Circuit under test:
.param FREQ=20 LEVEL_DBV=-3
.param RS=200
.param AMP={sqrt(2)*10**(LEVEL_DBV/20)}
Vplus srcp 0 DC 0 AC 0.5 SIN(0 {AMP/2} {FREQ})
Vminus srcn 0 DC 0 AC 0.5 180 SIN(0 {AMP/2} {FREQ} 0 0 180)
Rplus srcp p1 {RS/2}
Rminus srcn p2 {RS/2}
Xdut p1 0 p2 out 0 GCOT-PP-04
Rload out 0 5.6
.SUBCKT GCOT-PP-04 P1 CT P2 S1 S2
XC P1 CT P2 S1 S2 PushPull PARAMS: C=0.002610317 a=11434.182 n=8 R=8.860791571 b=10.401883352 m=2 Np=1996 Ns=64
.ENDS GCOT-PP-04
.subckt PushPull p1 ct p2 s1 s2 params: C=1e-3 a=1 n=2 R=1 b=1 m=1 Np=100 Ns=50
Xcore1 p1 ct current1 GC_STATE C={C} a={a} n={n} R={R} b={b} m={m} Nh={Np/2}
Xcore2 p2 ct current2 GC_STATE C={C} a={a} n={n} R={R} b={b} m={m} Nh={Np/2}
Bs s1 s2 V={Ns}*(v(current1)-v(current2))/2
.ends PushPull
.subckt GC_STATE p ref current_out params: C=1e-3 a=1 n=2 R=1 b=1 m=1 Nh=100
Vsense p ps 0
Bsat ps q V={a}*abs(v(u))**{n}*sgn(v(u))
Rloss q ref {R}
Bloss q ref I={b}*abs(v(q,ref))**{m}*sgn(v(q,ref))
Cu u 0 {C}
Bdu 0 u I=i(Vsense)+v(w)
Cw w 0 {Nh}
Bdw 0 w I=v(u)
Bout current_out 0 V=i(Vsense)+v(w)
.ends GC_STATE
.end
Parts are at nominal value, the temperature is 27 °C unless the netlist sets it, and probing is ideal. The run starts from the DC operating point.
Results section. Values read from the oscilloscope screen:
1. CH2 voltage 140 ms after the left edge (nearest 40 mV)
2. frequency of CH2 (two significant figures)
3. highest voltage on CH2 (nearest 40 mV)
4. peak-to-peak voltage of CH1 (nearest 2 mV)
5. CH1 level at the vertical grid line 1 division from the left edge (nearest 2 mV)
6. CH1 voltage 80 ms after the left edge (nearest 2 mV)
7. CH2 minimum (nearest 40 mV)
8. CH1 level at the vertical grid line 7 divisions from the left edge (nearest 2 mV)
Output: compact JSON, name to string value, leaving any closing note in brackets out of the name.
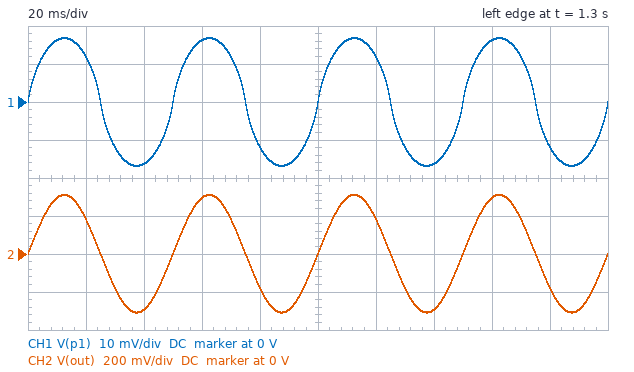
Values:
{"CH2 voltage 140 ms after the left edge": "-280 mV", "frequency of CH2": "20 Hz", "highest voltage on CH2": "320 mV", "peak-to-peak voltage of CH1": "34 mV", "CH1 level at the vertical grid line 1 division from the left edge": "12 mV", "CH1 voltage 80 ms after the left edge": "-12 mV", "CH2 minimum": "-320 mV", "CH1 level at the vertical grid line 7 divisions from the left edge": "-16 mV"}
